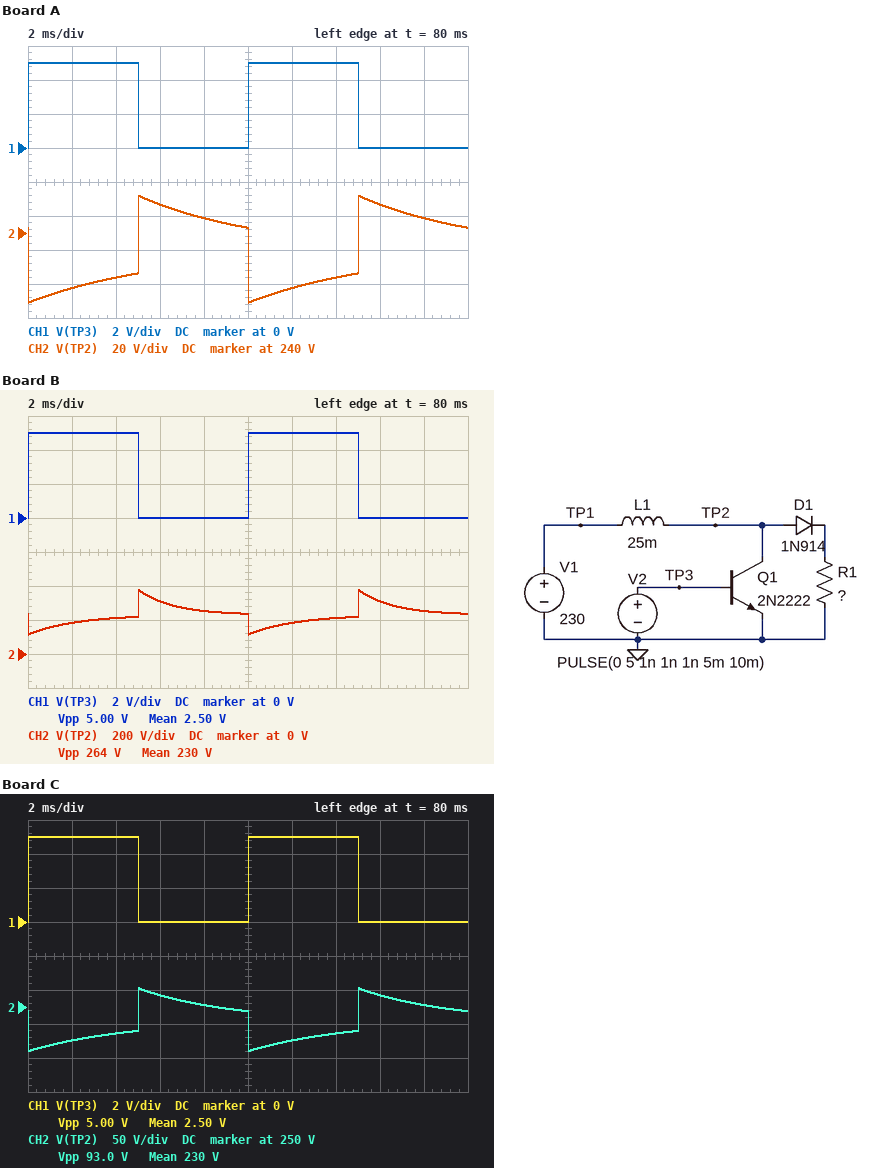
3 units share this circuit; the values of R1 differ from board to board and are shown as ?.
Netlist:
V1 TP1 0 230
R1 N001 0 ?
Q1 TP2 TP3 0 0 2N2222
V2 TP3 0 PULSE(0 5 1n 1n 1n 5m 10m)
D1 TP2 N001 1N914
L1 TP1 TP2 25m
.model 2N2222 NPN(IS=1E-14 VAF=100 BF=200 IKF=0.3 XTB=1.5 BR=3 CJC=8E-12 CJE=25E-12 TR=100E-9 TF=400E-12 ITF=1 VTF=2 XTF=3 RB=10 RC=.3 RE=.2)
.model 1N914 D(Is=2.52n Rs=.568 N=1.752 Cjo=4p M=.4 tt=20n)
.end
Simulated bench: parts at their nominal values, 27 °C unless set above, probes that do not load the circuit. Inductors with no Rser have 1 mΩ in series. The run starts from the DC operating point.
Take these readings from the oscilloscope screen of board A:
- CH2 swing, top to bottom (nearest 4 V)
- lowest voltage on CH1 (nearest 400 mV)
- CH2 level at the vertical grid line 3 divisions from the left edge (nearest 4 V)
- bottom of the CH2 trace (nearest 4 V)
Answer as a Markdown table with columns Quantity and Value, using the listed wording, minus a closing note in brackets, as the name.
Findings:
| Quantity | Value |
|---|---|
| CH2 swing, top to bottom | 64 V |
| lowest voltage on CH1 | 0 V |
| CH2 level at the vertical grid line 3 divisions from the left edge | 256 V |
| bottom of the CH2 trace | 200 V |
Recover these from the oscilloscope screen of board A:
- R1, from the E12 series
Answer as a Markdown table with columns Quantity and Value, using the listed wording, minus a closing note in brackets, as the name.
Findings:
| Quantity | Value |
|---|---|
| R1, from the E12 series | 3.9 Ω |
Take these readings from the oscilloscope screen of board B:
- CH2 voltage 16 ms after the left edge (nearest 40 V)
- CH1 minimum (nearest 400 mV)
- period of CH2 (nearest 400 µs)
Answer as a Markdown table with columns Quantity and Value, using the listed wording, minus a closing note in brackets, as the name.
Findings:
| Quantity | Value |
|---|---|
| CH2 voltage 16 ms after the left edge | 320 V |
| CH1 minimum | 0 V |
| period of CH2 | 10.0 ms |
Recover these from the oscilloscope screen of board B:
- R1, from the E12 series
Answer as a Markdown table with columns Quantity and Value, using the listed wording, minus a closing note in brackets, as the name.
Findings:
| Quantity | Value |
|---|---|
| R1, from the E12 series | 15 Ω |
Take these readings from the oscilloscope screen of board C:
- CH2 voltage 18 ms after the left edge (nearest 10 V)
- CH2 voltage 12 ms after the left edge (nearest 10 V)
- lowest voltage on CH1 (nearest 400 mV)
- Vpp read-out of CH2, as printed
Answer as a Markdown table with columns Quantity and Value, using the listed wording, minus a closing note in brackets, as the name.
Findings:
| Quantity | Value |
|---|---|
| CH2 voltage 18 ms after the left edge | 250 V |
| CH2 voltage 12 ms after the left edge | 200 V |
| lowest voltage on CH1 | 0 V |
| Vpp read-out of CH2, as printed | 93.0 V |
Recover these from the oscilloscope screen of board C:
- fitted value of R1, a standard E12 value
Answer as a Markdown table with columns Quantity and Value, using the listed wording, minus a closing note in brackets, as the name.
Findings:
| Quantity | Value |
|---|---|
| fitted value of R1, a standard E12 value | 5.6 Ω |
